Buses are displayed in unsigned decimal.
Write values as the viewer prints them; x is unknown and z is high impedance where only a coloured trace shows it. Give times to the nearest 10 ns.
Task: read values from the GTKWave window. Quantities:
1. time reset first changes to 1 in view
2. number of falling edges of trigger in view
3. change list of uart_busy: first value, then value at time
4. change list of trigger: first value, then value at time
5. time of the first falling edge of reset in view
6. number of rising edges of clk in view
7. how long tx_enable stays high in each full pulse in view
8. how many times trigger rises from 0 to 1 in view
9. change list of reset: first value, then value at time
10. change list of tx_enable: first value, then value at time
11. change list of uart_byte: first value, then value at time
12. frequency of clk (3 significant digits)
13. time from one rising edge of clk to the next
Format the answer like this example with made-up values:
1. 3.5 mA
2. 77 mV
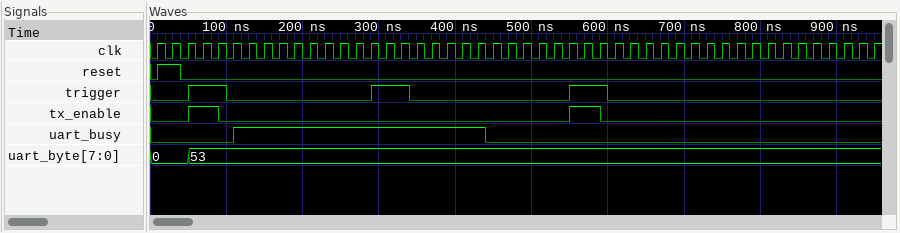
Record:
1. 10 ns
2. 3
3. 0, 1 at 110 ns, 0 at 440 ns
4. 0, 1 at 50 ns, 0 at 100 ns, 1 at 290 ns, 0 at 340 ns, 1 at 550 ns, 0 at 600 ns
5. 40 ns
6. 48
7. 40 ns, 40 ns
8. 3
9. 0, 1 at 10 ns, 0 at 40 ns
10. 0, 1 at 50 ns, 0 at 90 ns, 1 at 550 ns, 0 at 590 ns
11. 0, 53 at 50 ns
12. 50.0 MHz
13. 20 ns
